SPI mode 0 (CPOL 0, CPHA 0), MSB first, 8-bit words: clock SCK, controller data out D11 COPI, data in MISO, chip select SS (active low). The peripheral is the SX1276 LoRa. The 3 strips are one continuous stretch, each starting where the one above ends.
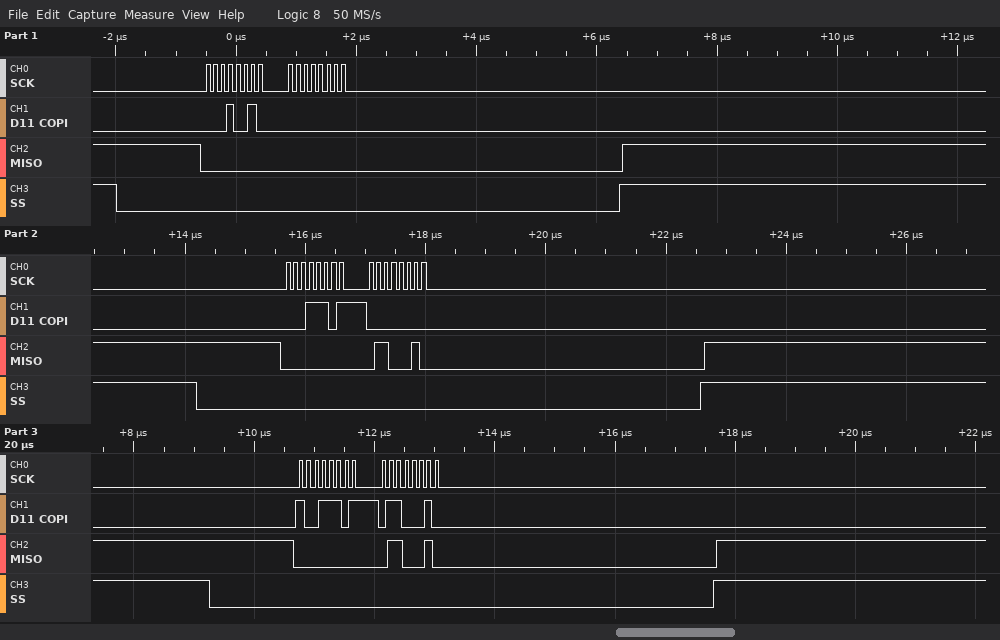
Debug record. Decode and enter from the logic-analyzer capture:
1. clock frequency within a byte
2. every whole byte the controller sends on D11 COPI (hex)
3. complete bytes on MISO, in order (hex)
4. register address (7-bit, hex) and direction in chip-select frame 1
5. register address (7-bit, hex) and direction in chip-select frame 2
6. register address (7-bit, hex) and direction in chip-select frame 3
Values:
8 MHz
12 00 1D 00 9D 62
00 00 00 62 00 62
0x12 read
0x1D read
0x1D write
